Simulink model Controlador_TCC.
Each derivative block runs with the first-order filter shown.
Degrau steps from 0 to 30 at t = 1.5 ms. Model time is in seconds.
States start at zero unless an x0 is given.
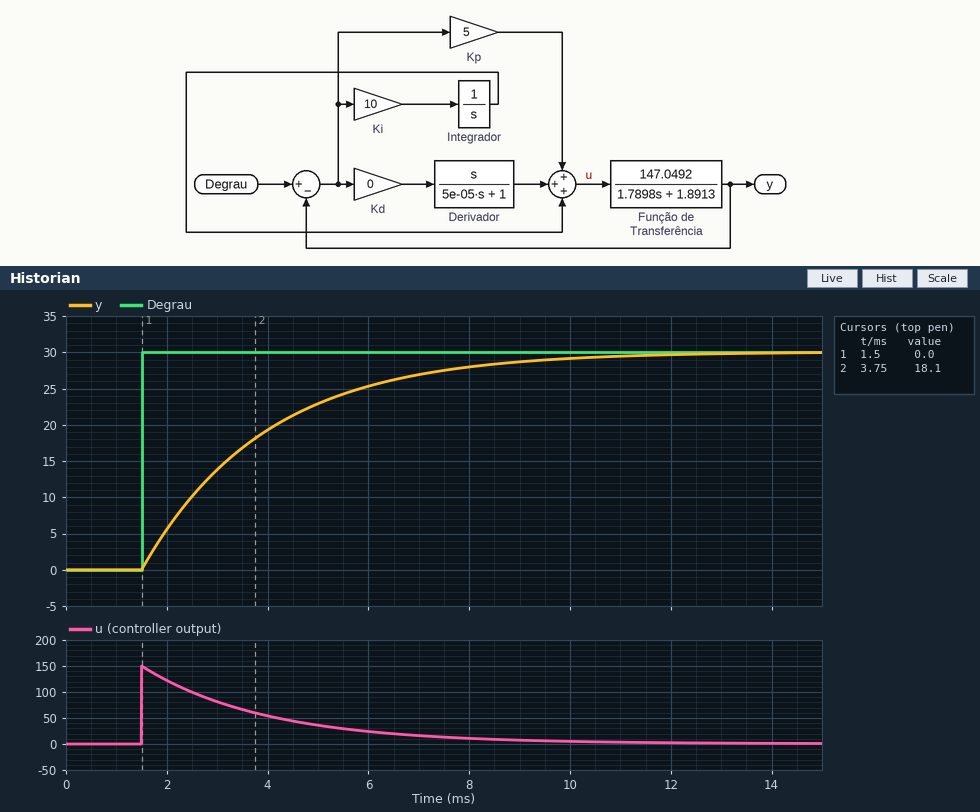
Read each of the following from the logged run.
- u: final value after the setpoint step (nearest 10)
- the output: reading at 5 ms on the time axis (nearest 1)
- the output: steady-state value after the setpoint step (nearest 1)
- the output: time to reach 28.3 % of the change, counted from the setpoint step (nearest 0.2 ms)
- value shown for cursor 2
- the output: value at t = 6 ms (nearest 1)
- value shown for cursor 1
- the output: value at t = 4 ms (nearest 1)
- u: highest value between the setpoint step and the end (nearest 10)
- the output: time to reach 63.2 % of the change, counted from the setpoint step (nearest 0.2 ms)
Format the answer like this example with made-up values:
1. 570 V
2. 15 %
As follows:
1. 0
2. 23
3. 30
4. 0.8 ms
5. 18.1
6. 25
7. 0.0
8. 19
9. 150
10. 2.4 ms
